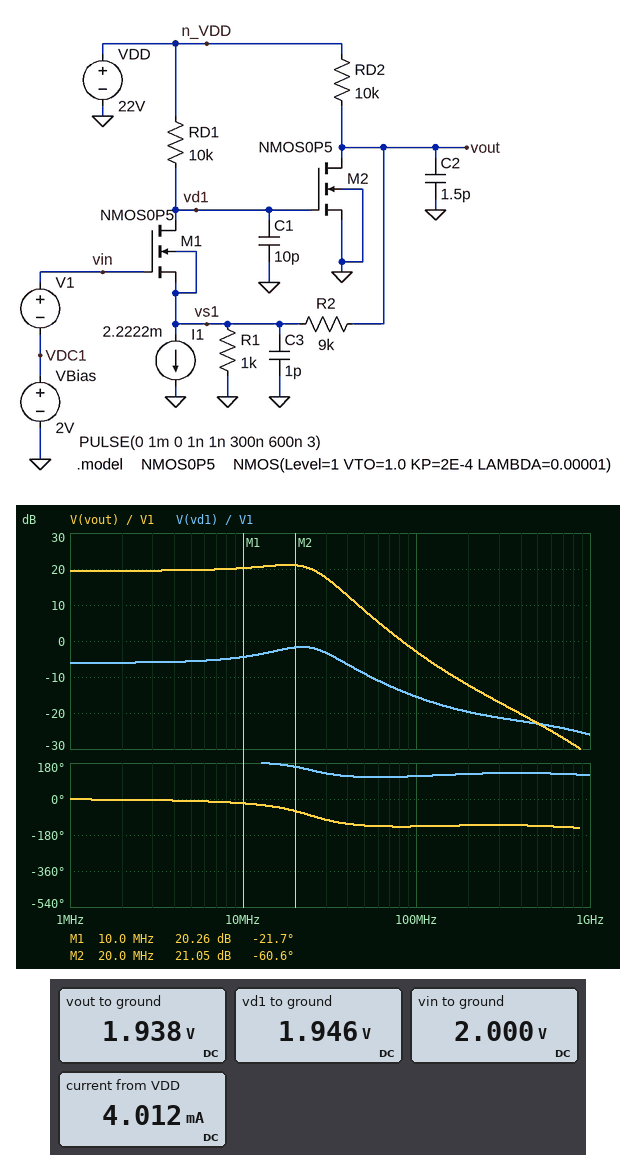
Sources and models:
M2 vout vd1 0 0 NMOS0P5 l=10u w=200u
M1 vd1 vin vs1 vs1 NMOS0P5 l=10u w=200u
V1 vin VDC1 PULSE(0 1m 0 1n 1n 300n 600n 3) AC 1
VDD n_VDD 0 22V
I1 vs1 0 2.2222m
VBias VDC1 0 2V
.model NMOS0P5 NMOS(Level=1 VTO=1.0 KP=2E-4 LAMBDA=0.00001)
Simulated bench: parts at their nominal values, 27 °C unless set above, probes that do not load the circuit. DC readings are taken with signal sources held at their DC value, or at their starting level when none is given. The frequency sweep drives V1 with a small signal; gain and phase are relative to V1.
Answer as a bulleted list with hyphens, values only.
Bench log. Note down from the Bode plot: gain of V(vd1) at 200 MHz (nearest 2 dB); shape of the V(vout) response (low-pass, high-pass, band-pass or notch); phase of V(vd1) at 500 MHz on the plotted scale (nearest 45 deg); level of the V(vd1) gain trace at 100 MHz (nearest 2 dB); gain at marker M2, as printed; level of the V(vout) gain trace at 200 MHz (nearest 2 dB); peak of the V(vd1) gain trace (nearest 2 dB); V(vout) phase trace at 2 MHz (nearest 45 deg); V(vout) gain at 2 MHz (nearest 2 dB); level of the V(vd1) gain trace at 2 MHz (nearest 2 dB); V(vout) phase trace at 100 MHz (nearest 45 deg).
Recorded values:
- -20 dB
- low-pass
- 135 deg
- -16 dB
- 21.05 dB
- -12 dB
- -2 dB
- 0 deg
- 20 dB
- -6 dB
- -135 deg
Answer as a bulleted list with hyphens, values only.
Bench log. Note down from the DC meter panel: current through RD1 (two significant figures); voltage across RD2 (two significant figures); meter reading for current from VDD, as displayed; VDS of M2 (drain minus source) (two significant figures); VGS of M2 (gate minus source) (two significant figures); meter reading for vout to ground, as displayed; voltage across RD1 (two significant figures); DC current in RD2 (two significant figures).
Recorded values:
- 2.0 mA
- 20 V
- 4.012 mA
- 1.9 V
- 1.9 V
- 1.938 V
- 20 V
- 2.0 mA
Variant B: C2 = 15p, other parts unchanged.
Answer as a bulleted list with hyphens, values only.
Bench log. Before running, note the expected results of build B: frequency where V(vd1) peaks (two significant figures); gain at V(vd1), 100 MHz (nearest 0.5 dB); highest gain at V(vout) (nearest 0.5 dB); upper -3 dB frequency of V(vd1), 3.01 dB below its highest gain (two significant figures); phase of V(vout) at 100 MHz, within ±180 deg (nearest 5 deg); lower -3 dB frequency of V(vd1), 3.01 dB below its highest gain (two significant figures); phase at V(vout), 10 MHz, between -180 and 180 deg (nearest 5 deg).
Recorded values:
- 7.7 MHz
- -16.0 dB
- 26.0 dB
- 9.7 MHz
- -150 deg
- 6.0 MHz
- -135 deg
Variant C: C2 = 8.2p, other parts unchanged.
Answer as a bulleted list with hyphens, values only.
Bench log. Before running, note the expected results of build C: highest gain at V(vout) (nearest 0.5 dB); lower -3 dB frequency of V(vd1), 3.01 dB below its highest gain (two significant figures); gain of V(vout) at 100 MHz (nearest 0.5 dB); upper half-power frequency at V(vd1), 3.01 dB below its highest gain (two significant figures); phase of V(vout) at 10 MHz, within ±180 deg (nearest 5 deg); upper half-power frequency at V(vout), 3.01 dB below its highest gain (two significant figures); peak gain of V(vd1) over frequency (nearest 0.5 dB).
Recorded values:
- 25.5 dB
- 7.8 MHz
- -18.0 dB
- 13 MHz
- -80 deg
- 12 MHz
- 8.5 dB
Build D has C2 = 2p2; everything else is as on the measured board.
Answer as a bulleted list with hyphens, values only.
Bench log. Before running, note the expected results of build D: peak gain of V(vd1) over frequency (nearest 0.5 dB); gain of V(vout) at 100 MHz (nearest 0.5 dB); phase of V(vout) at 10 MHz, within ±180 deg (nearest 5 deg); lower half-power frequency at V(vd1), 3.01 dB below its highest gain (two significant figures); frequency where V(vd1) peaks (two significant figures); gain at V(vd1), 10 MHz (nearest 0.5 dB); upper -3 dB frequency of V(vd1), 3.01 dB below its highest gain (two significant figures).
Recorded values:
- 0.5 dB
- -6.5 dB
- -25 deg
- 11 MHz
- 19 MHz
- -3.0 dB
- 28 MHz
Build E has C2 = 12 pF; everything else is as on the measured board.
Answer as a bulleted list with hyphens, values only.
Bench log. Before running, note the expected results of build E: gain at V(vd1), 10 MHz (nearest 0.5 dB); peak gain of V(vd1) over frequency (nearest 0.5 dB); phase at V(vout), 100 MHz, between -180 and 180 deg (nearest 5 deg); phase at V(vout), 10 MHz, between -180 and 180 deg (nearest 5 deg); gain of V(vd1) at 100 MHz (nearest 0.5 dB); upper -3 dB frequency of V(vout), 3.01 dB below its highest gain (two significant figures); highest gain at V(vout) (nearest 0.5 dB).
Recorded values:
- 9.0 dB
- 10.5 dB
- -150 deg
- -120 deg
- -16.0 dB
- 10 MHz
- 26.0 dB
